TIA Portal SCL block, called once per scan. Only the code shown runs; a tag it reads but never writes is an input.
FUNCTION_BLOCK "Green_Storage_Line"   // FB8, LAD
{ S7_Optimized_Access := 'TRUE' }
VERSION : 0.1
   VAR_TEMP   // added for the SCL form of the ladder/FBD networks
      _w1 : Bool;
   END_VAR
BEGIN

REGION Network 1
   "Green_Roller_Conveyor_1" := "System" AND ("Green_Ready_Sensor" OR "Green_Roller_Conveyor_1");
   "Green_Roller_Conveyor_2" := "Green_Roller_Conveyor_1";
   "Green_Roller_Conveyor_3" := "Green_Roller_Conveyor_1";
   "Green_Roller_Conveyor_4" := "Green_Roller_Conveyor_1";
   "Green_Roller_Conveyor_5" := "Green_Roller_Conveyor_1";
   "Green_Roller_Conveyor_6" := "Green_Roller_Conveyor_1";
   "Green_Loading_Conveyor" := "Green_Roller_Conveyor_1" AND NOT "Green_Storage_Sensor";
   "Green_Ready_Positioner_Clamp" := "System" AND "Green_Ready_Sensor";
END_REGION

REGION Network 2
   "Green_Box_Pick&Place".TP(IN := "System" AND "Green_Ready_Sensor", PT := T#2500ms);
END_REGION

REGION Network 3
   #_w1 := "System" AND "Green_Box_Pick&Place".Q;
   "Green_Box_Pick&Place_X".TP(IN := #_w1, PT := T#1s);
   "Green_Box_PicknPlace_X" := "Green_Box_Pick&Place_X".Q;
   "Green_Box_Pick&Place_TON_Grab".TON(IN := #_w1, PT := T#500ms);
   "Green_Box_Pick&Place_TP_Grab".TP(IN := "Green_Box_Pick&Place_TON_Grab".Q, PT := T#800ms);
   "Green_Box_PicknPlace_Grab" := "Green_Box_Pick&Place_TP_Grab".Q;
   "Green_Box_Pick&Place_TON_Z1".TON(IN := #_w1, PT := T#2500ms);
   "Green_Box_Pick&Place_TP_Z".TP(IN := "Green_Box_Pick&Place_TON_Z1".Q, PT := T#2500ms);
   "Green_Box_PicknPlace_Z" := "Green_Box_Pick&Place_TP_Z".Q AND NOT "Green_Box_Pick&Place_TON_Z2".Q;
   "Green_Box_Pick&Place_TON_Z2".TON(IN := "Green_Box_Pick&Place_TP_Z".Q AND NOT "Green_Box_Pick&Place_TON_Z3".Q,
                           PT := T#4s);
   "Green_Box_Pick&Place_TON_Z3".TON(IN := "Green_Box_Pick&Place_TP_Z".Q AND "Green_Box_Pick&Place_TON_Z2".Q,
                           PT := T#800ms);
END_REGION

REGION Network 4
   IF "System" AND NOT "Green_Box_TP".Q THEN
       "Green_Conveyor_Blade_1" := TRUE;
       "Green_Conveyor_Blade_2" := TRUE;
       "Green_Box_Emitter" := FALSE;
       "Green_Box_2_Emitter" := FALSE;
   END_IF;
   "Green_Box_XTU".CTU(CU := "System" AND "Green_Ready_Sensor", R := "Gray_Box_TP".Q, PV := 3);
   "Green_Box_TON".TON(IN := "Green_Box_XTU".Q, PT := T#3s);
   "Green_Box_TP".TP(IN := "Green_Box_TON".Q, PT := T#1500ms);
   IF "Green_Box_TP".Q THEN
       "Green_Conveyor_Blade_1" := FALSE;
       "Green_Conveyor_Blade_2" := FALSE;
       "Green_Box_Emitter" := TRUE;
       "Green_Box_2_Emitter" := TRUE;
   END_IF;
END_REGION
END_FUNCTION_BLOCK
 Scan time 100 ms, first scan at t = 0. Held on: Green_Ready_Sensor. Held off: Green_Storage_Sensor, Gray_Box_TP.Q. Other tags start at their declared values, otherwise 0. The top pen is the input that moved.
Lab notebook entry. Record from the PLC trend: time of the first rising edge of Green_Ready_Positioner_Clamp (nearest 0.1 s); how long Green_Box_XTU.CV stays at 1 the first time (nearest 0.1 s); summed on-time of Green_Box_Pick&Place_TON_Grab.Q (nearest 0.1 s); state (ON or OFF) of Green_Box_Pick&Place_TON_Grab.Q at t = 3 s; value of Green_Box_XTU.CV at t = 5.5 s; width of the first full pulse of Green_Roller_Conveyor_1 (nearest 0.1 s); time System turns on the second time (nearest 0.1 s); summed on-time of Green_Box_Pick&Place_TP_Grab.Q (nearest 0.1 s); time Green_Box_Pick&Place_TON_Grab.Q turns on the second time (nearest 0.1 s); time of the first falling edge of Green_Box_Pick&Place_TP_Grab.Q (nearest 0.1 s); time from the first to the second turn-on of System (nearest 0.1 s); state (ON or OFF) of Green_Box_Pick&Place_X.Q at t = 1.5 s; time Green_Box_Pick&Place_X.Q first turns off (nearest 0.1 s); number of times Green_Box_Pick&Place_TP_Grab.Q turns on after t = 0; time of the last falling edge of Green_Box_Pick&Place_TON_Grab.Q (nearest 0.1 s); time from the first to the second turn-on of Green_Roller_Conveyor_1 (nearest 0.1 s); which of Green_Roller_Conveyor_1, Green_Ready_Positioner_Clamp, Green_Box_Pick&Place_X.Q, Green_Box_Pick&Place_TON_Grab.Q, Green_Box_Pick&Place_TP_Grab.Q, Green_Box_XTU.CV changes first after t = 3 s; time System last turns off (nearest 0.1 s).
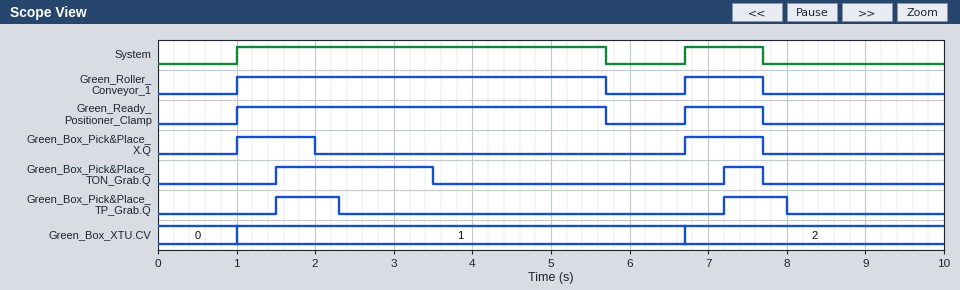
1.0 s
5.7 s
2.5 s
ON
1
4.7 s
6.7 s
1.6 s
7.2 s
2.3 s
5.7 s
ON
2.0 s
2
7.7 s
5.7 s
Green_Box_Pick&Place_TON_Grab.Q
7.7 s
